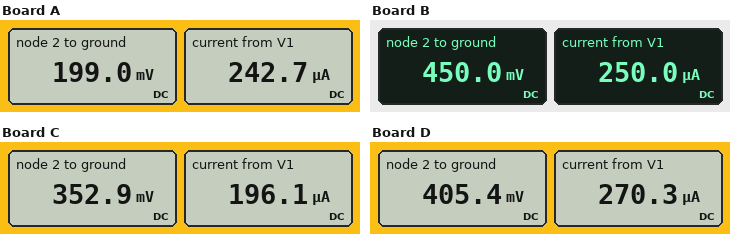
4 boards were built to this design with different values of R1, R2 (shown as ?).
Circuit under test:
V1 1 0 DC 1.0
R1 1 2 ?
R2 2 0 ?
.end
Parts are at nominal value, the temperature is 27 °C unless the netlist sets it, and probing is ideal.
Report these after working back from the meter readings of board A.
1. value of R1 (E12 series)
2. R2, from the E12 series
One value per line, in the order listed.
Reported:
3.3 kΩ
820 Ω
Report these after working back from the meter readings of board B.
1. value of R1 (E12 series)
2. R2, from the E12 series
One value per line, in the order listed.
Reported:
2.2 kΩ
1.8 kΩ
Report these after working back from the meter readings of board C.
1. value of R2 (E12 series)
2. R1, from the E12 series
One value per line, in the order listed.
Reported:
1.8 kΩ
3.3 kΩ
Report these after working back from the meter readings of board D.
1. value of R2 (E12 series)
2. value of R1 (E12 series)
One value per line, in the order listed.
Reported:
1.5 kΩ
2.2 kΩ
